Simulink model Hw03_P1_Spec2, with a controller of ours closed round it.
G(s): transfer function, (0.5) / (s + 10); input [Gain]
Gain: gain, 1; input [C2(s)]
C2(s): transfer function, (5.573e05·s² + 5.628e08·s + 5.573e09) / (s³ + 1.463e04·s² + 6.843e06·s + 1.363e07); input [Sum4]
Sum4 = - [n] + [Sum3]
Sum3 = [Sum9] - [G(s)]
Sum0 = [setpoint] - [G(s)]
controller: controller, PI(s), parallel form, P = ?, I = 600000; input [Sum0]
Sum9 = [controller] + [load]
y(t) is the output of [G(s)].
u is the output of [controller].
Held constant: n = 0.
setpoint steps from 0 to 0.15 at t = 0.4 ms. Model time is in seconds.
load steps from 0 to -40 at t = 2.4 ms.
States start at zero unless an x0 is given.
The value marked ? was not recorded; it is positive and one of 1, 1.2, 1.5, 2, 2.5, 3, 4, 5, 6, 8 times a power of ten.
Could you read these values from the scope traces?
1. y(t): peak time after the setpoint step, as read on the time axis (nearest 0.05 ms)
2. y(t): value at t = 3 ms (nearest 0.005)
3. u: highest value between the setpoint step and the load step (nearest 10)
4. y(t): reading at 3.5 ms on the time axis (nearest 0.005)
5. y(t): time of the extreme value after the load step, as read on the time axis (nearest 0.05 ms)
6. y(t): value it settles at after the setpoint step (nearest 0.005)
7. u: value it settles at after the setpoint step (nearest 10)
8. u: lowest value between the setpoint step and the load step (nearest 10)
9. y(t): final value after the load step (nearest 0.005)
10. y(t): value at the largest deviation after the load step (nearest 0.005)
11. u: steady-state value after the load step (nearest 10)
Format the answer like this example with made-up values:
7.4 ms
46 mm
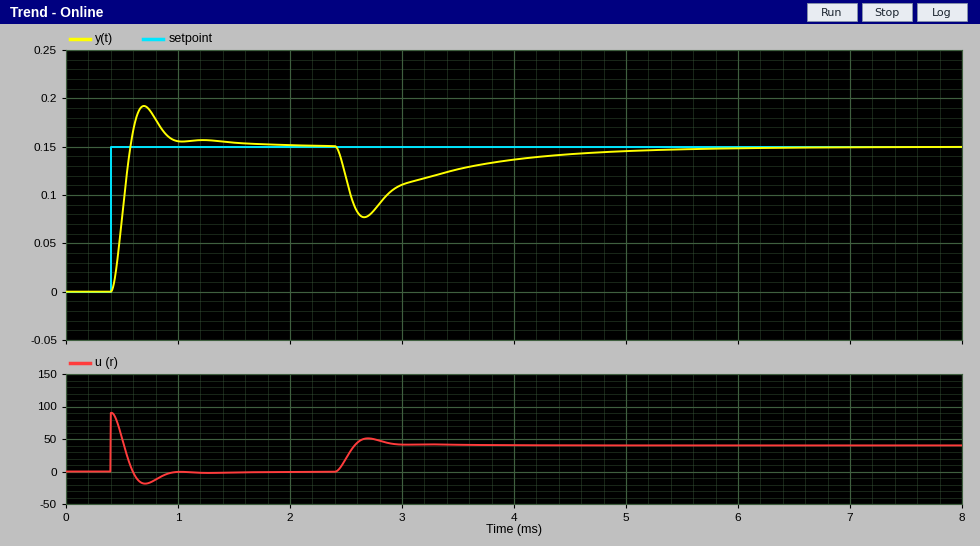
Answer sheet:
0.70 ms
0.110
90
0.125
2.65 ms
0.150
0
-20
0.150
0.075
40
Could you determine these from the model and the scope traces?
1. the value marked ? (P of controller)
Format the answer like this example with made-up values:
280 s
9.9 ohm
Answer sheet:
600
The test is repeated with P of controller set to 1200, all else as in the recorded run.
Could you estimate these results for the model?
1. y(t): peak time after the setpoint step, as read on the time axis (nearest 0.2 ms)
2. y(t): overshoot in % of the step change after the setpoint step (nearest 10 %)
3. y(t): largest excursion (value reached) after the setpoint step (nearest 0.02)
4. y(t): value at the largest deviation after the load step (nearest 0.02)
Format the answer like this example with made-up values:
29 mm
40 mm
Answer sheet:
0.6 ms
30 %
0.20
0.10
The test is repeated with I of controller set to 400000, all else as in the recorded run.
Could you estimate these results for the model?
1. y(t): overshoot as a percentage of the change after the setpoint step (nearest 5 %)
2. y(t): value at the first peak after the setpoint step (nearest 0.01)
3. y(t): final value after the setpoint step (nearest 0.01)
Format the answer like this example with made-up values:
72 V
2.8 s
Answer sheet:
25 %
0.19
0.15
